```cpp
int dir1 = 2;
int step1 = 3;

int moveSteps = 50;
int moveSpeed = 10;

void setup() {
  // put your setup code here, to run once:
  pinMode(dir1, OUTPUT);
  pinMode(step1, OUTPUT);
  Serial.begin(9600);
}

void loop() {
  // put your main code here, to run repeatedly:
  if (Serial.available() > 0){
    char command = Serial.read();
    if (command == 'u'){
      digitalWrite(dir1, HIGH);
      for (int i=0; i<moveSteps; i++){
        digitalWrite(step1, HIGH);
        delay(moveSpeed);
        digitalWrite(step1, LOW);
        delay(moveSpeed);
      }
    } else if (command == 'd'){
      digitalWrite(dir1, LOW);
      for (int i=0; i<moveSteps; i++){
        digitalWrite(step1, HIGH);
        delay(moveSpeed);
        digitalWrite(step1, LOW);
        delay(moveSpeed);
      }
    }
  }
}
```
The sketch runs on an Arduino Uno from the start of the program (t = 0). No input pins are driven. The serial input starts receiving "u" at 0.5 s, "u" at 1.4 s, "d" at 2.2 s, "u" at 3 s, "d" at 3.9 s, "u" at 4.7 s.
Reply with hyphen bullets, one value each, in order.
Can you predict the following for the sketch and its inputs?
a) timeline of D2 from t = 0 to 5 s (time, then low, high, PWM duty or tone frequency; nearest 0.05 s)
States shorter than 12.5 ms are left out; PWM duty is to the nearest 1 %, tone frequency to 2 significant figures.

- 0 s low; 0.5 s high; 2.5 s low; 3.5 s high; 4.5 s low
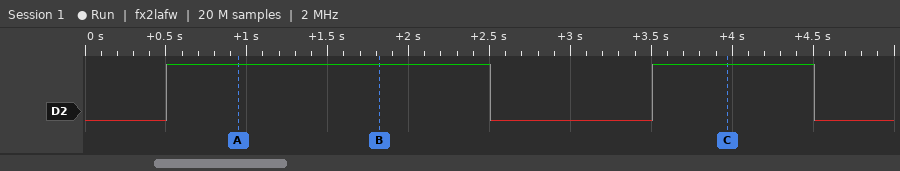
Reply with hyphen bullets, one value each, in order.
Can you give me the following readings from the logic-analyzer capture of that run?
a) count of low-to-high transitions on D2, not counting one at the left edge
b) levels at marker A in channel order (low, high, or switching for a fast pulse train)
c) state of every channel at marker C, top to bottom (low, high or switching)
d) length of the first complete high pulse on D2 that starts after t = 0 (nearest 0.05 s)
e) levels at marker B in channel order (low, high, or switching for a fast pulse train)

- 2
- D2 high
- D2 high
- 2.00 s
- D2 high
